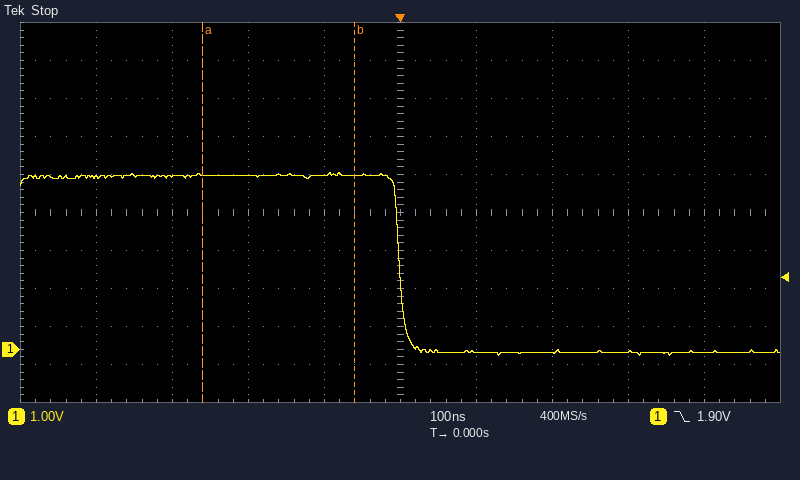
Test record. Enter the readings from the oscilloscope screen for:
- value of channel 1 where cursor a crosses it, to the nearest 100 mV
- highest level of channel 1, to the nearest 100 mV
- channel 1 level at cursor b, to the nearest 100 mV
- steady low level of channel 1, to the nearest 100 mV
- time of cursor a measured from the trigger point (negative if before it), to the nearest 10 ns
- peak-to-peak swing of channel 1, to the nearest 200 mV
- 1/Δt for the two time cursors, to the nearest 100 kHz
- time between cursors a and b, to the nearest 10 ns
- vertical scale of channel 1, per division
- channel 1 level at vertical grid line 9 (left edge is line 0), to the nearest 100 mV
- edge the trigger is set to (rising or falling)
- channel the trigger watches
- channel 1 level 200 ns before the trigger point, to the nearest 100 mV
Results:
4.6 V
4.7 V
4.6 V
-100 mV
-260 ns
4.8 V
5.0 MHz
200 ns
1 V
-100 mV
falling
channel 1
4.6 V
